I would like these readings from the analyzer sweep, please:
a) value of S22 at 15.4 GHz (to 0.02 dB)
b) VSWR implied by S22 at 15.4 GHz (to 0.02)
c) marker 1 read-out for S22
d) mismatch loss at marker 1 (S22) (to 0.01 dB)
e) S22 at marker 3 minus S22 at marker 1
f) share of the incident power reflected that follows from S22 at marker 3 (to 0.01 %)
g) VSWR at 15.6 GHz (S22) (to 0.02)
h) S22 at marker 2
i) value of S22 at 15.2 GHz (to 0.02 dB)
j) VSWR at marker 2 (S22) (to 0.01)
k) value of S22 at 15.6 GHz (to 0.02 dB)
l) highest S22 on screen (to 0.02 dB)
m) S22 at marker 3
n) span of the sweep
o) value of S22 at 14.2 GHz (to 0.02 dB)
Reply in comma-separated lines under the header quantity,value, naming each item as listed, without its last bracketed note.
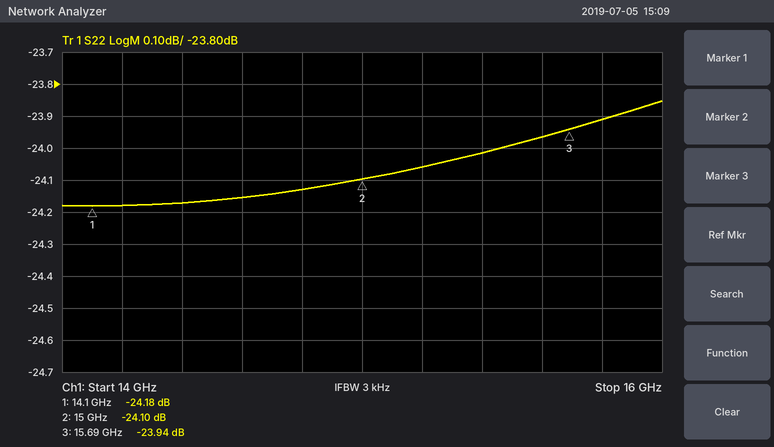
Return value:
quantity,value
value of S22 at 15.4 GHz,-24.02 dB
VSWR implied by S22 at 15.4 GHz,1.14
marker 1 read-out for S22,-24.18 dB
mismatch loss at marker 1 (S22),0.02 dB
S22 at marker 3 minus S22 at marker 1,0.24 dB
share of the incident power reflected that follows from S22 at marker 3,0.40 %
VSWR at 15.6 GHz (S22),1.14
S22 at marker 2,-24.10 dB
value of S22 at 15.2 GHz,-24.06 dB
VSWR at marker 2 (S22),1.13
value of S22 at 15.6 GHz,-23.96 dB
highest S22 on screen,-23.86 dB
S22 at marker 3,-23.94 dB
span of the sweep,2 GHz
value of S22 at 14.2 GHz,-24.18 dB
